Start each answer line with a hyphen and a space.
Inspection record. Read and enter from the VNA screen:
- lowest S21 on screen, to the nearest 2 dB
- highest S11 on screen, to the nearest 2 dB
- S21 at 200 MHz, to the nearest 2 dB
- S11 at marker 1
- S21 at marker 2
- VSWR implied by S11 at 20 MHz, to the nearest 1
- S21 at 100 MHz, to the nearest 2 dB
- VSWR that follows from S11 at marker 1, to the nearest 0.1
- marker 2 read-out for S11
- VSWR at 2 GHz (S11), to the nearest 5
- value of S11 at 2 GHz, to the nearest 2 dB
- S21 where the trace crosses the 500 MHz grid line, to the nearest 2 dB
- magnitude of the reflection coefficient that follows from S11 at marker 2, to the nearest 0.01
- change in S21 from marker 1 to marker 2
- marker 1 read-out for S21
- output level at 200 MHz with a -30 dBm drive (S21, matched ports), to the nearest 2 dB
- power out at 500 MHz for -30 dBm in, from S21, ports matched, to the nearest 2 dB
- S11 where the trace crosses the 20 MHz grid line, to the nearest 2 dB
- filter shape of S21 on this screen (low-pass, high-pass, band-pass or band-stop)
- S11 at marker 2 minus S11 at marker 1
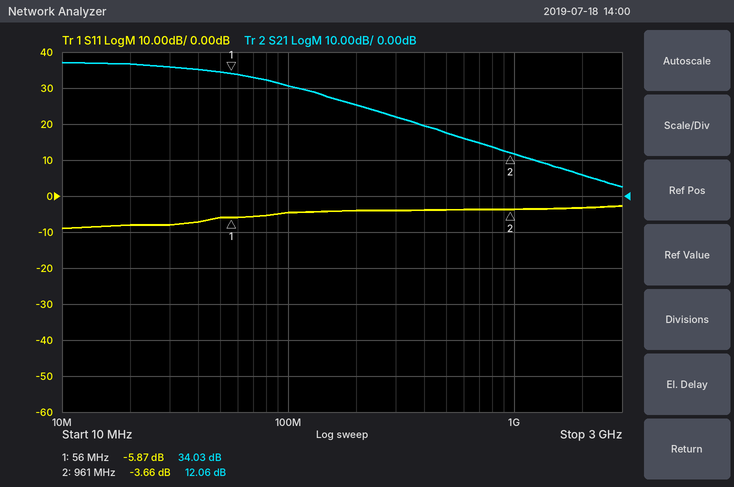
- 2 dB
- -2 dB
- 26 dB
- -5.87 dB
- 12.06 dB
- 2
- 30 dB
- 3.1
- -3.66 dB
- 5
- -4 dB
- 18 dB
- 0.66
- -21.97 dB
- 34.03 dB
- -4 dBm
- -12 dBm
- -8 dB
- low-pass
- 2.21 dB
